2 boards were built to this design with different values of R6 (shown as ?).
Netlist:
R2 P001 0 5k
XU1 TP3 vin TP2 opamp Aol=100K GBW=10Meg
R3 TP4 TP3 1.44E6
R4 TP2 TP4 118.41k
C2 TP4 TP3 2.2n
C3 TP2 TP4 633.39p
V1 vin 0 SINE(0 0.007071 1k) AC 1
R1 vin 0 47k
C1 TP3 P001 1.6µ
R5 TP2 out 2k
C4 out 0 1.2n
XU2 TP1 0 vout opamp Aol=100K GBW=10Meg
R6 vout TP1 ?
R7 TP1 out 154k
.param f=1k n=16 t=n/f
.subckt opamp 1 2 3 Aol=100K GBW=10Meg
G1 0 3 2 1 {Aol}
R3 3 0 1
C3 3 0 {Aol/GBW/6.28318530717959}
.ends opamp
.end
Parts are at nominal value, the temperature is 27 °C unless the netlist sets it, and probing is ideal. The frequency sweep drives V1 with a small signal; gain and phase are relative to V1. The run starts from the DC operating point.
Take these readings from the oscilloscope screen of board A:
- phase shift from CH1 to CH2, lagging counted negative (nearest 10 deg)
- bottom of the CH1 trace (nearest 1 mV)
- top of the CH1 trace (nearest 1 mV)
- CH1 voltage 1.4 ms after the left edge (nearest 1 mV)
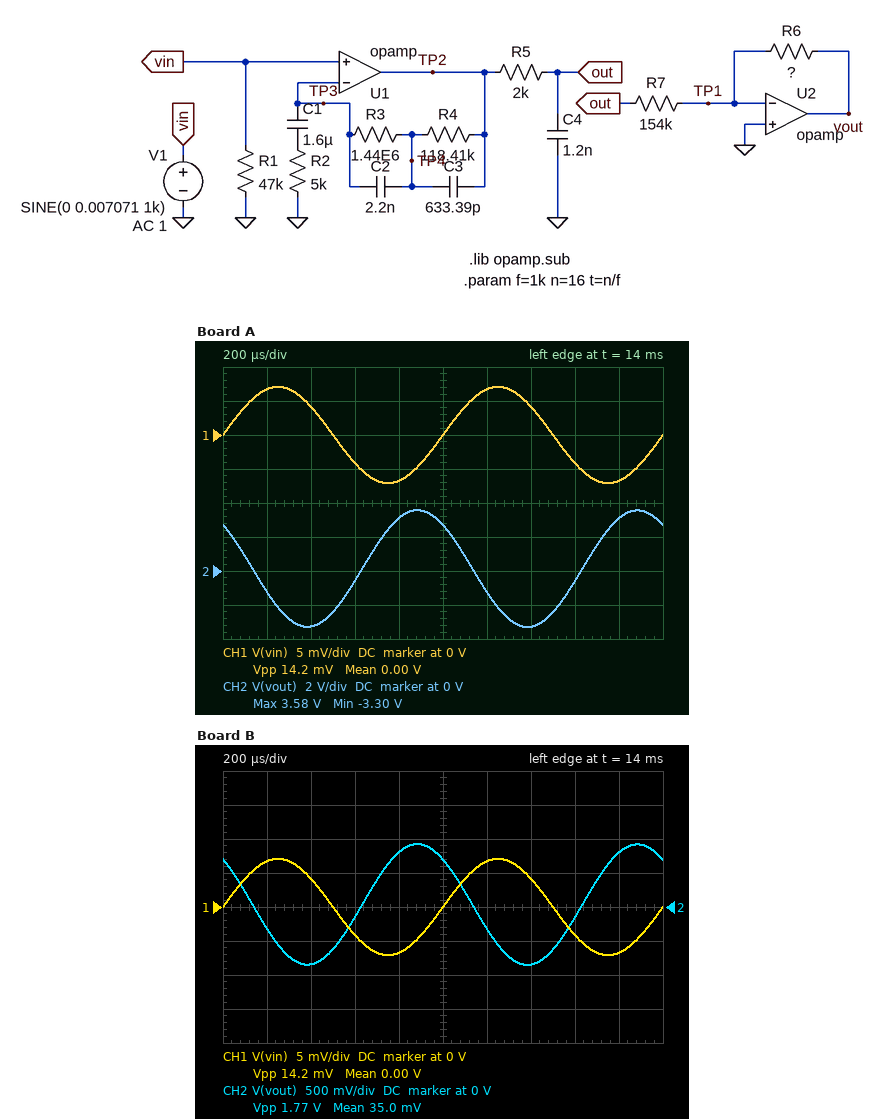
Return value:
130 deg
-7 mV
7 mV
4 mV
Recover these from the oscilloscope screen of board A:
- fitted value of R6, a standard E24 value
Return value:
2.4 MΩ
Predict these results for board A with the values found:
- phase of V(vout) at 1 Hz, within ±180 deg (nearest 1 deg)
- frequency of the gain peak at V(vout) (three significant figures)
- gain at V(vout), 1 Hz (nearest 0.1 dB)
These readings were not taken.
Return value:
-98 deg
31.7 Hz
47.7 dB
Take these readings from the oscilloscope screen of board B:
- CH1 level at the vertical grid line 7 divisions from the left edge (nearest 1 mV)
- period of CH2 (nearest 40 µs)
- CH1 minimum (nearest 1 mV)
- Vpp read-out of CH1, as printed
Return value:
4 mV
1.00 ms
-7 mV
14.2 mV
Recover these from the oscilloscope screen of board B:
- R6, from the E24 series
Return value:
620 kΩ
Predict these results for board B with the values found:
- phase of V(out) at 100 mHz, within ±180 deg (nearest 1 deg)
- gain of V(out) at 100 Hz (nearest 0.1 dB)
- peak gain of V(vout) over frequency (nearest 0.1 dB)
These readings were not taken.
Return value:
57 deg
42.8 dB
59.0 dB
